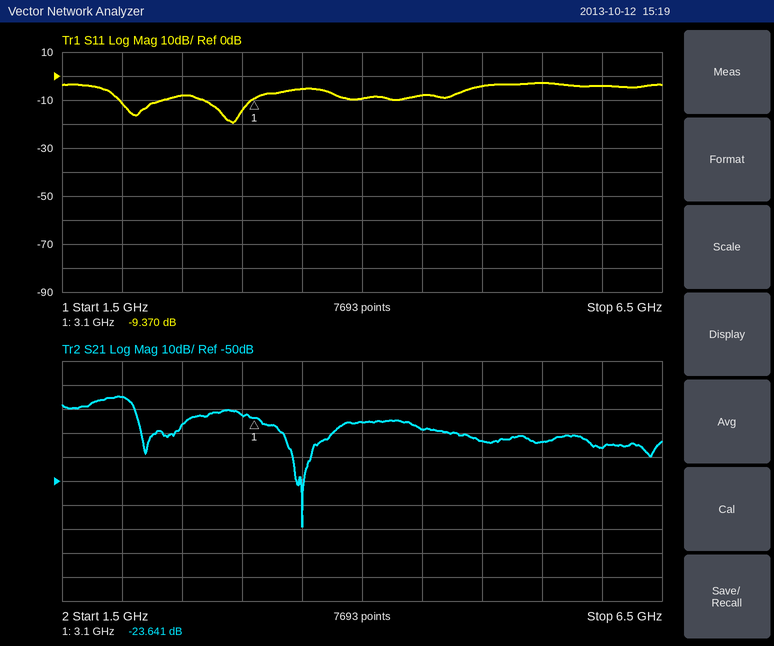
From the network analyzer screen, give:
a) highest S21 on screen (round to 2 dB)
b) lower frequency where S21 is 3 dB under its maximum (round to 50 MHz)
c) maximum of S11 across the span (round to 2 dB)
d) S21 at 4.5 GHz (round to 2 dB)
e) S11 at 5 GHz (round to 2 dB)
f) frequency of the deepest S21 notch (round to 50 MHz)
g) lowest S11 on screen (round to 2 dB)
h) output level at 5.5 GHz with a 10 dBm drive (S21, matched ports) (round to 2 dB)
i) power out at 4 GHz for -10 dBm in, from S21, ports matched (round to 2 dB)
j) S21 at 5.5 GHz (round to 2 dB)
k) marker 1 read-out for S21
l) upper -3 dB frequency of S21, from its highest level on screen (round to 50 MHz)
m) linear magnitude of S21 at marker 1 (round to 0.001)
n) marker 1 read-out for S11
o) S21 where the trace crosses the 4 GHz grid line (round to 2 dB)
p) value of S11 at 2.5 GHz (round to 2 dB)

-14 dB
1.75 GHz
-2 dB
-28 dB
-4 dB
3.50 GHz
-20 dB
-24 dBm
-36 dBm
-34 dB
-23.641 dB
2.10 GHz
0.066
-9.370 dB
-26 dB
-8 dB
